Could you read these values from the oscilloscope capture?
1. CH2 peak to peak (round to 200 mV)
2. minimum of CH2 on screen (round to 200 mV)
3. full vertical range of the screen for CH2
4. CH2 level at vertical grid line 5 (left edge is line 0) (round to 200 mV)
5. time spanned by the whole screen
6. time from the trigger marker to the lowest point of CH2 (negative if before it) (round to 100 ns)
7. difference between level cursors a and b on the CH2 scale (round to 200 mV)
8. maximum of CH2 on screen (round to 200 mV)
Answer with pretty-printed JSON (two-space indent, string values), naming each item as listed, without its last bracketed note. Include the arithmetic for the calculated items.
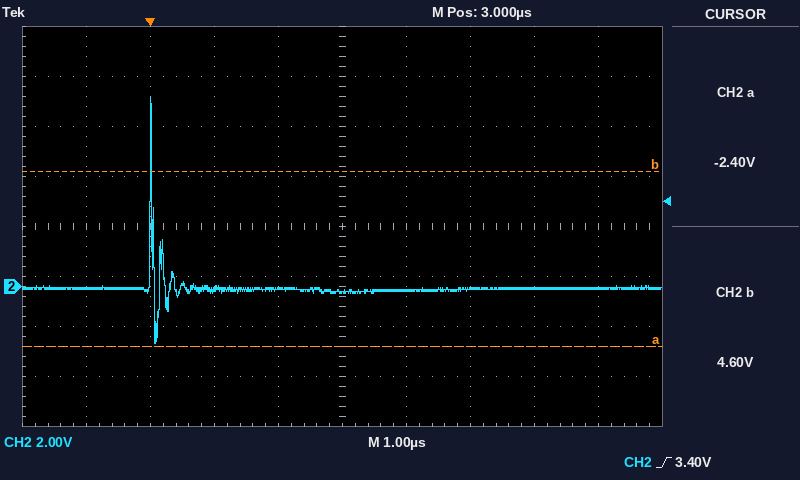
{
  "CH2 peak to peak": "7.6 V − (-2.2 V) = 9.8 V",
  "minimum of CH2 on screen": "-2.2 V",
  "full vertical range of the screen for CH2": "16 V",
  "CH2 level at vertical grid line 5 (left edge is line 0)": "-200 mV",
  "time spanned by the whole screen": "10 µs",
  "time from the trigger marker to the lowest point of CH2 (negative if before it)": "+100 ns",
  "difference between level cursors a and b on the CH2 scale": "7.0 V",
  "maximum of CH2 on screen": "7.6 V"
}
